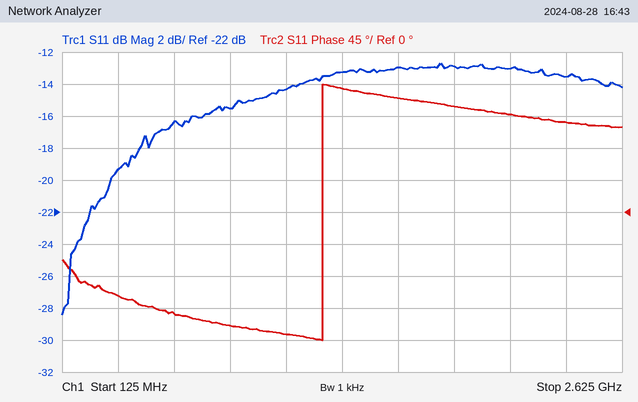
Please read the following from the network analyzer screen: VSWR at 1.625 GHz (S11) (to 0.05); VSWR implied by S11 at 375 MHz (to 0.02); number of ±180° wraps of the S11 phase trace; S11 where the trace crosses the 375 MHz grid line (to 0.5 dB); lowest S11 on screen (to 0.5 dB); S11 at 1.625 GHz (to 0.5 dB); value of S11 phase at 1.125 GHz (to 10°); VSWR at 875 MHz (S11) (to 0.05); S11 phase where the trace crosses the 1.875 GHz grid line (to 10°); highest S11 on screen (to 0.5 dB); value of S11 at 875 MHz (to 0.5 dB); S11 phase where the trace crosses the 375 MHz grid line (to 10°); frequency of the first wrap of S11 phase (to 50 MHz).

1.60
1.24
1
-19.5 dB
-28.5 dB
-13.0 dB
-170°
1.40
150°
-12.5 dB
-15.5 dB
-120°
1.30 GHz
